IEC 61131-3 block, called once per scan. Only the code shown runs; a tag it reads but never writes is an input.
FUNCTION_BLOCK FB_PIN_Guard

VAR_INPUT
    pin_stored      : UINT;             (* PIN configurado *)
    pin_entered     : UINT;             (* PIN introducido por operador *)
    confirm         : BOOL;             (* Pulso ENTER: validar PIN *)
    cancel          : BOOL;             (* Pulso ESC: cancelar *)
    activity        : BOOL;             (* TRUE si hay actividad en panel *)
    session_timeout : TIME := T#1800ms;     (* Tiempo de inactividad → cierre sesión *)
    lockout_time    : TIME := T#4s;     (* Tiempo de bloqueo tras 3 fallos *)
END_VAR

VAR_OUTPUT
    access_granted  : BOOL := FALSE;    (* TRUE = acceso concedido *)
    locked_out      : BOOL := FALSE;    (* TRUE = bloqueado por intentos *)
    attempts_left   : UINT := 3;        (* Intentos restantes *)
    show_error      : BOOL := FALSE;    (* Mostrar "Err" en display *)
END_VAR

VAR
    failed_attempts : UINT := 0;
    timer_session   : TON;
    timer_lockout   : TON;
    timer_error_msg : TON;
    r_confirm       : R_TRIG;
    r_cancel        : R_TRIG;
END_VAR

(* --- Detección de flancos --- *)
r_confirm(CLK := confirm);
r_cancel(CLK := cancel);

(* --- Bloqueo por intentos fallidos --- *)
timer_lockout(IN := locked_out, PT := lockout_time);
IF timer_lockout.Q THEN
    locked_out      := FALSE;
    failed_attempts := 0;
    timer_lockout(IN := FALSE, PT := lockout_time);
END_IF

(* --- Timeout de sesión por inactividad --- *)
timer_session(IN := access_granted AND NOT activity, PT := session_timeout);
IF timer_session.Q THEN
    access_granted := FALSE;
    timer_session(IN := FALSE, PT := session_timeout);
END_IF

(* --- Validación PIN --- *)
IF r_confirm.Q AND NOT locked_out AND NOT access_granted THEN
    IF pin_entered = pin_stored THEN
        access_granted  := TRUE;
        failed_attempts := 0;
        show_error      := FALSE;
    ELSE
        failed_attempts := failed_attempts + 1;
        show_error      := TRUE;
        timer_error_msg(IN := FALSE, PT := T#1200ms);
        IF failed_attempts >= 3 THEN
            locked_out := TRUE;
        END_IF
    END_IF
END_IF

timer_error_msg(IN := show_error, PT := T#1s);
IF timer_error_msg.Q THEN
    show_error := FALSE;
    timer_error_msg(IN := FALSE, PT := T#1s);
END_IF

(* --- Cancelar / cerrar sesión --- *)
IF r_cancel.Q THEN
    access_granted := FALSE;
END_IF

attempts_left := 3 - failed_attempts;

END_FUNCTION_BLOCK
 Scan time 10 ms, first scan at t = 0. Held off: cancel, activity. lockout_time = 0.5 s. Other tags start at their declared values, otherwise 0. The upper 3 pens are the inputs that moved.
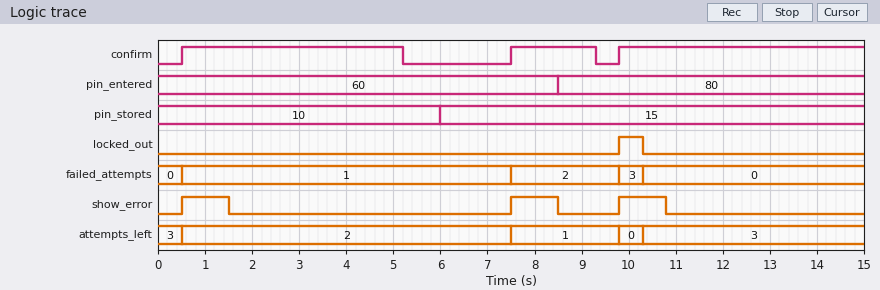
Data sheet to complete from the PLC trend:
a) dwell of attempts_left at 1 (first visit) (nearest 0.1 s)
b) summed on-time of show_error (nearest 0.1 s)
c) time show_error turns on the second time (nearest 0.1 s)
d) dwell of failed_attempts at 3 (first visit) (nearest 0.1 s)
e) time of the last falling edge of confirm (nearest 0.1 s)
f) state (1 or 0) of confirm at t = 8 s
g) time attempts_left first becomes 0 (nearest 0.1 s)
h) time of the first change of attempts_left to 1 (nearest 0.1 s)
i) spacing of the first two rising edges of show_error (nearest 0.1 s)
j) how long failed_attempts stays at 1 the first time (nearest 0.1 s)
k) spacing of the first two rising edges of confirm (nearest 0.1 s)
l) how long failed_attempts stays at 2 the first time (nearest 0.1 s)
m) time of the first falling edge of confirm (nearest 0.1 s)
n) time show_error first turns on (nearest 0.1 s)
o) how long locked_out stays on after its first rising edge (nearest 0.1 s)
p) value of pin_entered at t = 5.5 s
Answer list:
2.3 s
3.0 s
7.5 s
0.5 s
9.3 s
1
9.8 s
7.5 s
7.0 s
7.0 s
7.0 s
2.3 s
5.2 s
0.5 s
0.5 s
60
